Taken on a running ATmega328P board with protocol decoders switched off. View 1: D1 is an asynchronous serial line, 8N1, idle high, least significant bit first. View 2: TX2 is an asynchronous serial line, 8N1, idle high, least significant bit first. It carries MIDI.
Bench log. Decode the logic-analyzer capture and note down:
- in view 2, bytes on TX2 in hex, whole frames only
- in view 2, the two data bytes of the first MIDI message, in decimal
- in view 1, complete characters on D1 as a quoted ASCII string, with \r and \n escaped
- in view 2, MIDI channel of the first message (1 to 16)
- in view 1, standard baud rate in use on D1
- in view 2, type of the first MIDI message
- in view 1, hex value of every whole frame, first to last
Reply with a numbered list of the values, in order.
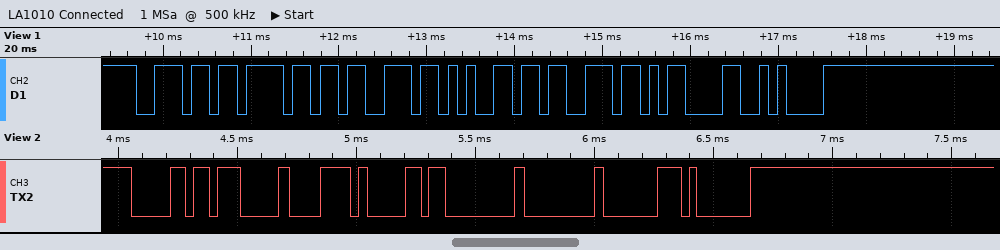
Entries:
1. B0 07 78 B0 00 00 C0 01
2. 7, 120
3. "noses\r\n"
4. 1
5. 9600 baud
6. Control Change
7. 0x6E 0x6F 0x73 0x65 0x73 0x0D 0x0A
